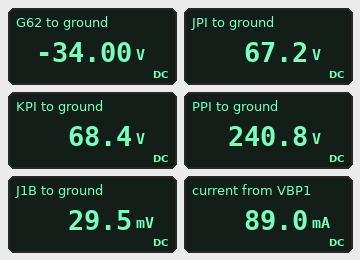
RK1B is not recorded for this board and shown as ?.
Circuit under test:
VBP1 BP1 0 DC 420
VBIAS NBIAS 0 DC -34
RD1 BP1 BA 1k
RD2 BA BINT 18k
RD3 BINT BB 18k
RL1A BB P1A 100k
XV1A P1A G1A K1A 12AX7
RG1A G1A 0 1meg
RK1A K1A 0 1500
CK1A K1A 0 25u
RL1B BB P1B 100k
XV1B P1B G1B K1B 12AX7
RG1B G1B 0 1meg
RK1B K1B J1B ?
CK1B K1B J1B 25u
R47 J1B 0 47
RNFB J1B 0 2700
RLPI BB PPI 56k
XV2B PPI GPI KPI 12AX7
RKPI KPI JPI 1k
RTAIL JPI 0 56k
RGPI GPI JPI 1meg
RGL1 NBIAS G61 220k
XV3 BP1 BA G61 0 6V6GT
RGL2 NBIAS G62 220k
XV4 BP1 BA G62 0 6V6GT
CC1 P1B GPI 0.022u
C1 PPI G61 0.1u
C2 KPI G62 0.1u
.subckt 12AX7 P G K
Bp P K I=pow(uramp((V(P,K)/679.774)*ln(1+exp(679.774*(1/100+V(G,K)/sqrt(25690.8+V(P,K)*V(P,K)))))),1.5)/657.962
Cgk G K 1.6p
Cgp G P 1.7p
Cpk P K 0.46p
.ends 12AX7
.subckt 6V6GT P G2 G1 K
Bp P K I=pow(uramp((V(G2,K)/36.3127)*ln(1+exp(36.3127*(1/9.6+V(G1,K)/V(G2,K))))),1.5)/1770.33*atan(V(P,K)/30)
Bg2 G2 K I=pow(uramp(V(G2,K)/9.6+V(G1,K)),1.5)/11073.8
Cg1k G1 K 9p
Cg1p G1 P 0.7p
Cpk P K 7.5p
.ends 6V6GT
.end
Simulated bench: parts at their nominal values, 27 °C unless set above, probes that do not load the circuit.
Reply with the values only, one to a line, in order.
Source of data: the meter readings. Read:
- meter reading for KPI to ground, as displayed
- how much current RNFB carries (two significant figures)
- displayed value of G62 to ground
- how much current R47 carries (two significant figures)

68.4 V
11 µA
-34.00 V
630 µA
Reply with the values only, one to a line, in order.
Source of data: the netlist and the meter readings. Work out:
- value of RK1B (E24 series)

3.6 kΩ
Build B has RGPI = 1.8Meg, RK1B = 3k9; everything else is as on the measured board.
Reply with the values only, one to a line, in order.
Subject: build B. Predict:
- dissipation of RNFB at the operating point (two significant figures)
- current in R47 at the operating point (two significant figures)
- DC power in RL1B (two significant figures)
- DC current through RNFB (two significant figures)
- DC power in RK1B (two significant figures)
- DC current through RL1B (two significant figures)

290 nW
600 µA
37 mW
10 µA
1.4 mW
610 µA
